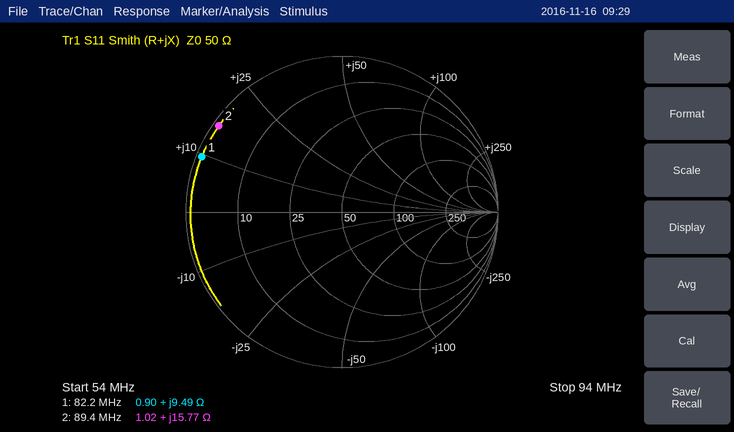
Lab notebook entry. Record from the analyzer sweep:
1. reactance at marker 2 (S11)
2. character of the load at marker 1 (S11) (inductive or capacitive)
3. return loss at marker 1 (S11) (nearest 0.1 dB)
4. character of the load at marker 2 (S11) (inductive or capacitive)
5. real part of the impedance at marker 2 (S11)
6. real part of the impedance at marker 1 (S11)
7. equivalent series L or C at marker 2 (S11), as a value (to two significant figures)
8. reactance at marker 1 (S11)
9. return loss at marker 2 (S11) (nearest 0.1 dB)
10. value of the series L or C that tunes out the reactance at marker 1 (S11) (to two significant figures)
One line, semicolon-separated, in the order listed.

+15.77 Ω; inductive; 0.3 dB; inductive; 1.02 Ω; 0.90 Ω; 28 nH; +9.49 Ω; 0.3 dB; 200 pF
